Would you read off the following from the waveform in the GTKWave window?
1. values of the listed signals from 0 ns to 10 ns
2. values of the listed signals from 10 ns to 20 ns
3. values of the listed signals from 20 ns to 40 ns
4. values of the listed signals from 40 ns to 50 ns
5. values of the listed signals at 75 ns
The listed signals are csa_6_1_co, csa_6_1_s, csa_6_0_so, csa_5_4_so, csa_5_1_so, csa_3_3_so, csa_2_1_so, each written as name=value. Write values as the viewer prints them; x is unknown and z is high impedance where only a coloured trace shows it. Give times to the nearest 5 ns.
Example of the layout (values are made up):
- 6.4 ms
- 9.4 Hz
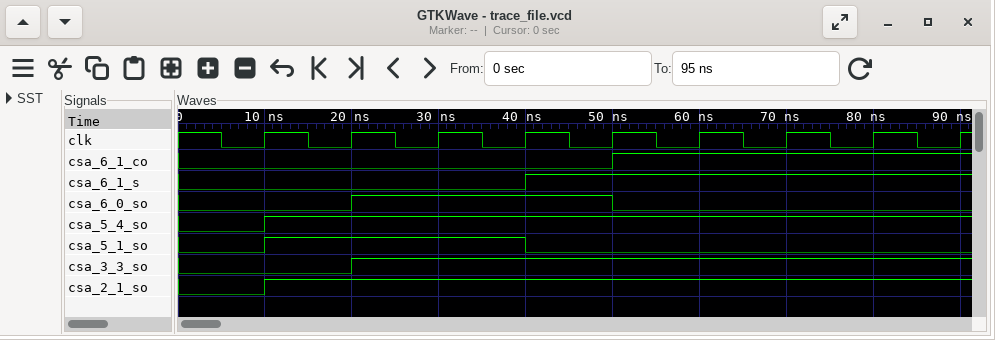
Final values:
- csa_6_1_co=0, csa_6_1_s=0, csa_6_0_so=0, csa_5_4_so=0, csa_5_1_so=0, csa_3_3_so=0, csa_2_1_so=0
- csa_6_1_co=0, csa_6_1_s=0, csa_6_0_so=0, csa_5_4_so=1, csa_5_1_so=1, csa_3_3_so=0, csa_2_1_so=1
- csa_6_1_co=0, csa_6_1_s=0, csa_6_0_so=1, csa_5_4_so=1, csa_5_1_so=1, csa_3_3_so=1, csa_2_1_so=1
- csa_6_1_co=0, csa_6_1_s=1, csa_6_0_so=1, csa_5_4_so=1, csa_5_1_so=0, csa_3_3_so=1, csa_2_1_so=1
- csa_6_1_co=1, csa_6_1_s=1, csa_6_0_so=0, csa_5_4_so=1, csa_5_1_so=0, csa_3_3_so=1, csa_2_1_so=1
